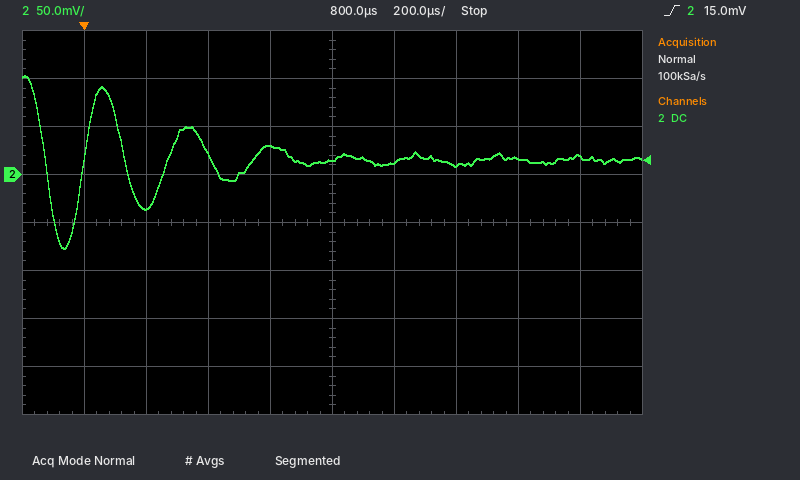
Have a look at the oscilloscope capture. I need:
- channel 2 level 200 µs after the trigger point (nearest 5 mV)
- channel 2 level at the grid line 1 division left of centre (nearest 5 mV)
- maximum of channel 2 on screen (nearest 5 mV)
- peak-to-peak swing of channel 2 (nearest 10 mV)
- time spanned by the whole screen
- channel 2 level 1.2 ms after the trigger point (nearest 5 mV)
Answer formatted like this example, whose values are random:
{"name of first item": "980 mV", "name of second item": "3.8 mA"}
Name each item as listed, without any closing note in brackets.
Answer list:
{"channel 2 level 200 µs after the trigger point": "-35 mV", "channel 2 level at the grid line 1 division left of centre": "30 mV", "maximum of channel 2 on screen": "105 mV", "peak-to-peak swing of channel 2": "180 mV", "time spanned by the whole screen": "2 ms", "channel 2 level 1.2 ms after the trigger point": "10 mV"}
